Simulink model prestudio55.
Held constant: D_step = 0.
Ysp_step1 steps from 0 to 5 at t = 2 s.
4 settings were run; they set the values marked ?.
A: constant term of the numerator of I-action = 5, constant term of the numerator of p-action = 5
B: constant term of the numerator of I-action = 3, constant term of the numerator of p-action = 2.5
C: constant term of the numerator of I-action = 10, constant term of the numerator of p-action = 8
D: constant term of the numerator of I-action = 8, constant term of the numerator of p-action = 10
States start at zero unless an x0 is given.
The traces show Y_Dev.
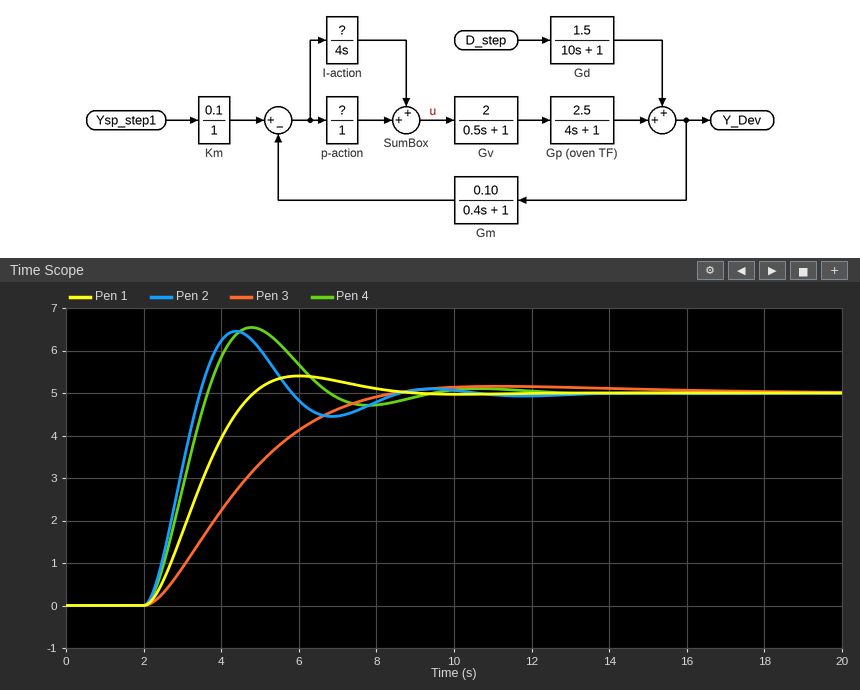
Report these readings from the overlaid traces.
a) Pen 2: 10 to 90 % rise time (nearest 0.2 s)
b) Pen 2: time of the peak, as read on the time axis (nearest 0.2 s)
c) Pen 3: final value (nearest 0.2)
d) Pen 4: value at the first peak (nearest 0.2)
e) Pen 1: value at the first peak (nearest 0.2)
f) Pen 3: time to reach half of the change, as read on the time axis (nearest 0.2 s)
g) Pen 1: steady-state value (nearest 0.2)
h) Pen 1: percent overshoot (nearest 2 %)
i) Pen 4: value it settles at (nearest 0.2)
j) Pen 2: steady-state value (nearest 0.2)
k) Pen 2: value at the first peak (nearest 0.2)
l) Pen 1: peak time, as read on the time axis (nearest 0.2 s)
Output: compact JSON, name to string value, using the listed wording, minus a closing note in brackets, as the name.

{"Pen 2: 10 to 90 % rise time": "1.0 s", "Pen 2: time of the peak, as read on the time axis": "4.4 s", "Pen 3: final value": "5.0", "Pen 4: value at the first peak": "6.6", "Pen 1: value at the first peak": "5.4", "Pen 3: time to reach half of the change, as read on the time axis": "4.2 s", "Pen 1: steady-state value": "5.0", "Pen 1: percent overshoot": "8 %", "Pen 4: value it settles at": "5.0", "Pen 2: steady-state value": "5.0", "Pen 2: value at the first peak": "6.4", "Pen 1: peak time, as read on the time axis": "6.0 s"}
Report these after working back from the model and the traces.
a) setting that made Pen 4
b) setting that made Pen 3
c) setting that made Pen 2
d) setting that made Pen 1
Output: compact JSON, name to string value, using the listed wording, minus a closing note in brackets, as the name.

{"setting that made Pen 4": "C", "setting that made Pen 3": "B", "setting that made Pen 2": "D", "setting that made Pen 1": "A"}
